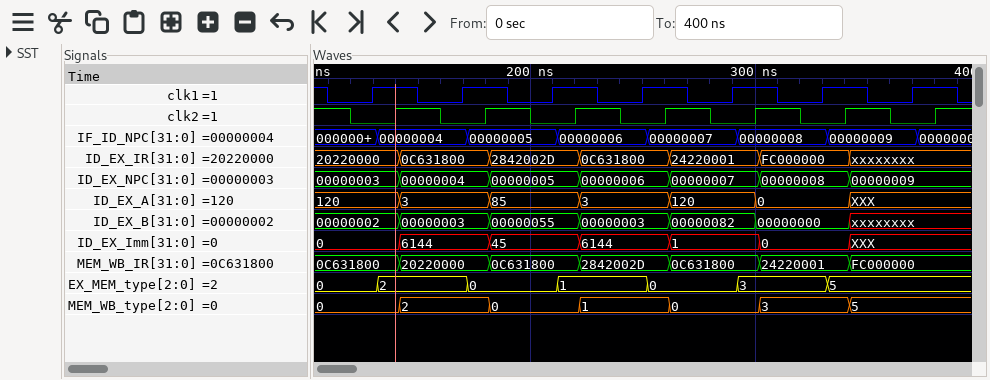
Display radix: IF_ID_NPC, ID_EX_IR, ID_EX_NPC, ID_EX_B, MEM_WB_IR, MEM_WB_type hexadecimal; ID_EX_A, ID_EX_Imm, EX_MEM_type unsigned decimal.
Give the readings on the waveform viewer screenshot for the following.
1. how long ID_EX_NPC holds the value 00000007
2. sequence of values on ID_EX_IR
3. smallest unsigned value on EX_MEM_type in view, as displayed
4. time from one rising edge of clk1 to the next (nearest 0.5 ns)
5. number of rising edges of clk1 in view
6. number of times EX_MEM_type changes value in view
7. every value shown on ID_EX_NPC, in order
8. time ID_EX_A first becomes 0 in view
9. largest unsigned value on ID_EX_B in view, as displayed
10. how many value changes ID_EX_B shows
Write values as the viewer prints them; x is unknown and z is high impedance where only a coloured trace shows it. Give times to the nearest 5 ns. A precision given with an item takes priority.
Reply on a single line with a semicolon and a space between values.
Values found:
40 ns; 20220000, 0C631800, 2842002D, 0C631800, 24220001, FC000000, xxxxxxxx; 0; 40 ns; 7; 6; 00000003, 00000004, 00000005, 00000006, 00000007, 00000008, 00000009; 300 ns; 00000082; 6
